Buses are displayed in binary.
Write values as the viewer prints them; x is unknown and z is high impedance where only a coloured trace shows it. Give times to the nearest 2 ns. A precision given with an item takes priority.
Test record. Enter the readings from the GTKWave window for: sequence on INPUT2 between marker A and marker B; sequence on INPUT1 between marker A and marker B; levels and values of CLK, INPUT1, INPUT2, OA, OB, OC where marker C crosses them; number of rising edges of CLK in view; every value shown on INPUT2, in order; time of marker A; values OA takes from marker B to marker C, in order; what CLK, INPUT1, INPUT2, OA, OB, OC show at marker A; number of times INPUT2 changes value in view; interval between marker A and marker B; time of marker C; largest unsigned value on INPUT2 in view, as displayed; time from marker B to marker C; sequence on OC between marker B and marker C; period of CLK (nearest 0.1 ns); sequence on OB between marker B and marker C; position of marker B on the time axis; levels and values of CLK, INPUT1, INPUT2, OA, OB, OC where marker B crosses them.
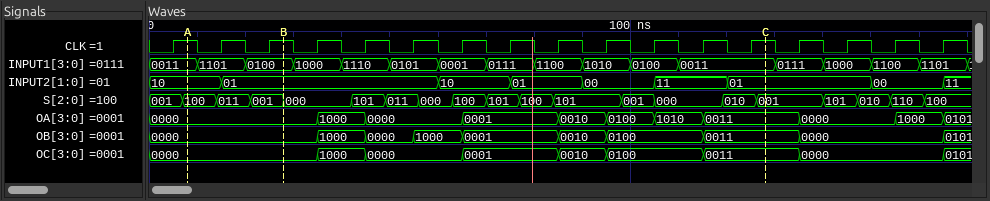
10, 01
0011, 1101, 0100
CLK=1, INPUT1=0011, INPUT2=01, OA=0011, OB=0011, OC=0011
17
10, 01, 10, 01, 00, 11, 01, 00, 11
8 ns
0000, 1000, 0000, 0001, 0010, 0100, 1010, 0011
CLK=1, INPUT1=0011, INPUT2=10, OA=0000, OB=0000, OC=0000
8
20 ns
128 ns
11
100 ns
0000, 1000, 0000, 0001, 0010, 0100, 0011
10 ns
0000, 1000, 0000, 1000, 0001, 0010, 0100, 0011
28 ns
CLK=1, INPUT1=0100, INPUT2=01, OA=0000, OB=0000, OC=0000
